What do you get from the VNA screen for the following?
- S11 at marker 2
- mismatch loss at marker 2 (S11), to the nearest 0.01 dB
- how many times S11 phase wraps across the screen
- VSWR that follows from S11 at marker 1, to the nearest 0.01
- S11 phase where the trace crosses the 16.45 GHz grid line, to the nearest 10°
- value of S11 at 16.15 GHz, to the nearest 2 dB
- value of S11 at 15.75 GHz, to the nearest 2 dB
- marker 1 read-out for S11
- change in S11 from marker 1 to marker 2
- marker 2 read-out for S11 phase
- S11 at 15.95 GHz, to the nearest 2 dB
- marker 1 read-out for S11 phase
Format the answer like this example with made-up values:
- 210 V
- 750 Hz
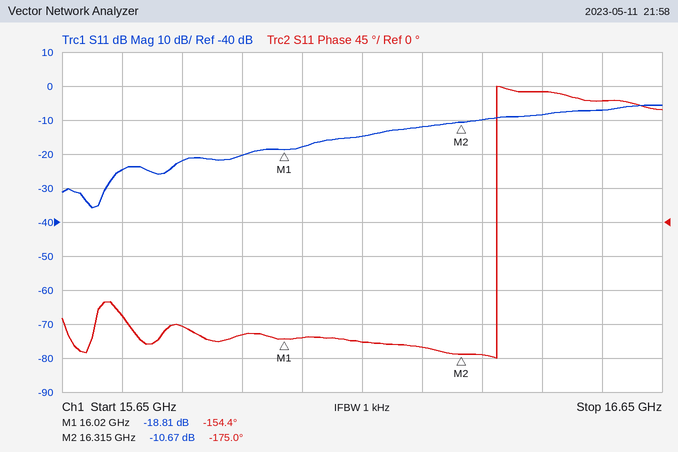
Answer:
- -10.67 dB
- 0.39 dB
- 1
- 1.26
- 170°
- -14 dB
- -24 dB
- -18.81 dB
- 8.14 dB
- -175.0°
- -20 dB
- -154.4°
